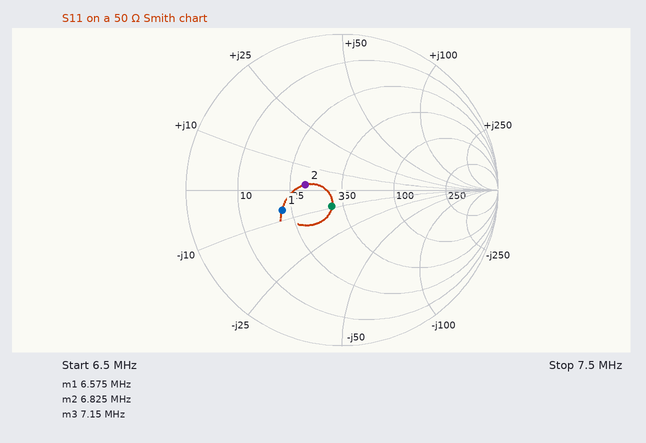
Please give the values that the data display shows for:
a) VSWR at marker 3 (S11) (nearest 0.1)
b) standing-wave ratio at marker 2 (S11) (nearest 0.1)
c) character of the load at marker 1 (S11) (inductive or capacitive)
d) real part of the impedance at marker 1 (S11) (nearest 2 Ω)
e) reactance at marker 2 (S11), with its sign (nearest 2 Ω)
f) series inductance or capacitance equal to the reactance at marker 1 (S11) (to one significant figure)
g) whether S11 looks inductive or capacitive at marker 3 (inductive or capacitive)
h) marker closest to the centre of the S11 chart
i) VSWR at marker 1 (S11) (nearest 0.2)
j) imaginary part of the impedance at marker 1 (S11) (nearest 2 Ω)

1.3
1.6
capacitive
22 Ω
+2 Ω
4 nF
capacitive
marker 3
2.4
-6 Ω
